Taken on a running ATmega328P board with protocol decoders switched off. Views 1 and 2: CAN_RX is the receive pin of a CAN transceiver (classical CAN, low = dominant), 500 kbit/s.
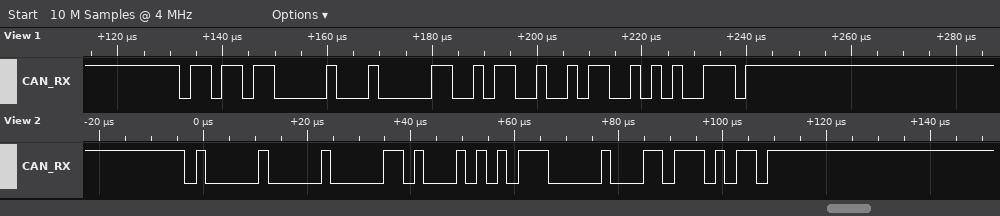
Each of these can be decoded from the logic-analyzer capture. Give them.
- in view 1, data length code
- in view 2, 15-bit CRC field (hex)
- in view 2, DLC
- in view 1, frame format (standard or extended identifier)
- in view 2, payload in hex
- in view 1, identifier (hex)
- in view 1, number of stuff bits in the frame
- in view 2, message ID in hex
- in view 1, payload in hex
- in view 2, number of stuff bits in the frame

2
0x0375
2
standard
8A B8
0x6D8
2
0x400
09 64
4
